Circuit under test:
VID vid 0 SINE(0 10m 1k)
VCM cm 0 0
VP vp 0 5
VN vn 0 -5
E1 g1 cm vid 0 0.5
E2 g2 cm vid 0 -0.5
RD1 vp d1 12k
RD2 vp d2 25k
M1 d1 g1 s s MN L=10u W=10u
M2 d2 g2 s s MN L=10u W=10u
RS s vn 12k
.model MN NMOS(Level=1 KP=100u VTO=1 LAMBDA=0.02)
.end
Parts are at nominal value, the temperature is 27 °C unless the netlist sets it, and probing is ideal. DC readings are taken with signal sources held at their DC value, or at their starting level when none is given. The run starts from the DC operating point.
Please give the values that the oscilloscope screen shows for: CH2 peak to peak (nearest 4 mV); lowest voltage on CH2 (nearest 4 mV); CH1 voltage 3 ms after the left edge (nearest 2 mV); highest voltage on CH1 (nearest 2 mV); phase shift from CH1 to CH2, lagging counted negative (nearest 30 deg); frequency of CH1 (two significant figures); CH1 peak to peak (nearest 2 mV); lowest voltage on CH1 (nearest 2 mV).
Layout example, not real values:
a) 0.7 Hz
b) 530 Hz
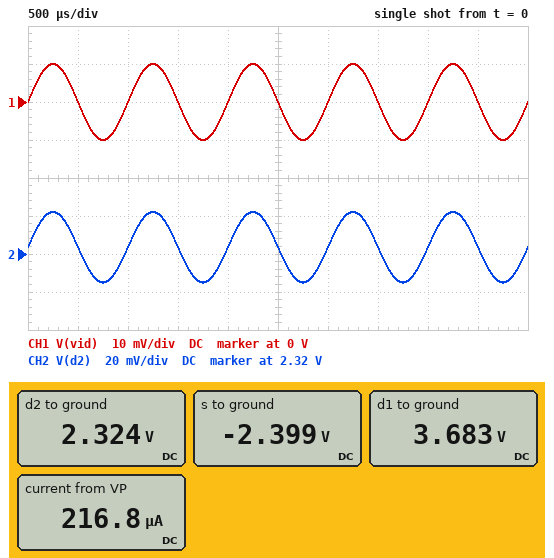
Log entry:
a) 36 mV
b) 2.304 V
c) 0 V
d) 10 mV
e) 0 deg
f) 1.0 kHz
g) 20 mV
h) -10 mV
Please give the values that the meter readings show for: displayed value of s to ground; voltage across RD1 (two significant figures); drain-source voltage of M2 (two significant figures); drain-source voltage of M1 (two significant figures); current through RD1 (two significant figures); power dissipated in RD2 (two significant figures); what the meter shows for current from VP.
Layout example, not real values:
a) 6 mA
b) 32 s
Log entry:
a) -2.399 V
b) 1.3 V
c) 4.7 V
d) 6.1 V
e) 110 µA
f) 290 µW
g) 216.8 µA
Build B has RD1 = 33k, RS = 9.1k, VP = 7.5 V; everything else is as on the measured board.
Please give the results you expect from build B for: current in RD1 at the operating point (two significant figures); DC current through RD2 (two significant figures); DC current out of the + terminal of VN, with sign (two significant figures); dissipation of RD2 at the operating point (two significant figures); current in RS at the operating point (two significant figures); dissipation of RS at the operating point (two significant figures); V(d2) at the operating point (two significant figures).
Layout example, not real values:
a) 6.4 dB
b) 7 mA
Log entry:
a) 130 µA
b) 140 µA
c) -270 µA
d) 460 µW
e) 270 µA
f) 660 µW
g) 4.1 V
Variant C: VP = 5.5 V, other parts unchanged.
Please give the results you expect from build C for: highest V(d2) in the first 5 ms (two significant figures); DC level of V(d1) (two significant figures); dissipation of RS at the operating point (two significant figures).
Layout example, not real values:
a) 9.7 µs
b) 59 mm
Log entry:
a) 2.8 V
b) 4.2 V
c) 570 µW
